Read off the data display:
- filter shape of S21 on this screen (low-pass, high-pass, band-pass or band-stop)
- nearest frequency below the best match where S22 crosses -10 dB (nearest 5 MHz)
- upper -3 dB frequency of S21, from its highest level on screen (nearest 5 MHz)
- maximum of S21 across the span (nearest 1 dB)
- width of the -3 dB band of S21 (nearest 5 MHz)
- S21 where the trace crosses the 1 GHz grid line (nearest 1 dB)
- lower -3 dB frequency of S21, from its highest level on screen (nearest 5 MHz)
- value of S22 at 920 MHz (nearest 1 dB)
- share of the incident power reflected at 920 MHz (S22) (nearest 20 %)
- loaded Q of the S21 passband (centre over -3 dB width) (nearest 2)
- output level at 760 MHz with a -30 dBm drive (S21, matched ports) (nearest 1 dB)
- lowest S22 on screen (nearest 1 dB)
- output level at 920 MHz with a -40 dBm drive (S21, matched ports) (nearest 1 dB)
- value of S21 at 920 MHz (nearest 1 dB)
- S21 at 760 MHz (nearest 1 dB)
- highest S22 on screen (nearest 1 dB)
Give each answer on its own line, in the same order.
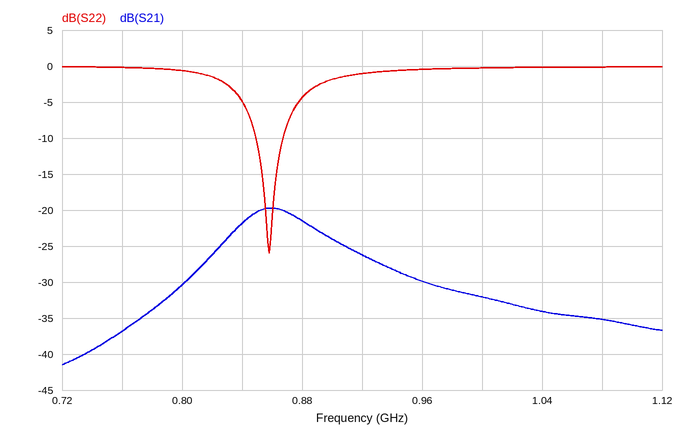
band-pass
850 MHz
890 MHz
-20 dB
55 MHz
-32 dB
835 MHz
-1 dB
80 %
16
-67 dBm
-26 dB
-66 dBm
-26 dB
-37 dB
0 dB
